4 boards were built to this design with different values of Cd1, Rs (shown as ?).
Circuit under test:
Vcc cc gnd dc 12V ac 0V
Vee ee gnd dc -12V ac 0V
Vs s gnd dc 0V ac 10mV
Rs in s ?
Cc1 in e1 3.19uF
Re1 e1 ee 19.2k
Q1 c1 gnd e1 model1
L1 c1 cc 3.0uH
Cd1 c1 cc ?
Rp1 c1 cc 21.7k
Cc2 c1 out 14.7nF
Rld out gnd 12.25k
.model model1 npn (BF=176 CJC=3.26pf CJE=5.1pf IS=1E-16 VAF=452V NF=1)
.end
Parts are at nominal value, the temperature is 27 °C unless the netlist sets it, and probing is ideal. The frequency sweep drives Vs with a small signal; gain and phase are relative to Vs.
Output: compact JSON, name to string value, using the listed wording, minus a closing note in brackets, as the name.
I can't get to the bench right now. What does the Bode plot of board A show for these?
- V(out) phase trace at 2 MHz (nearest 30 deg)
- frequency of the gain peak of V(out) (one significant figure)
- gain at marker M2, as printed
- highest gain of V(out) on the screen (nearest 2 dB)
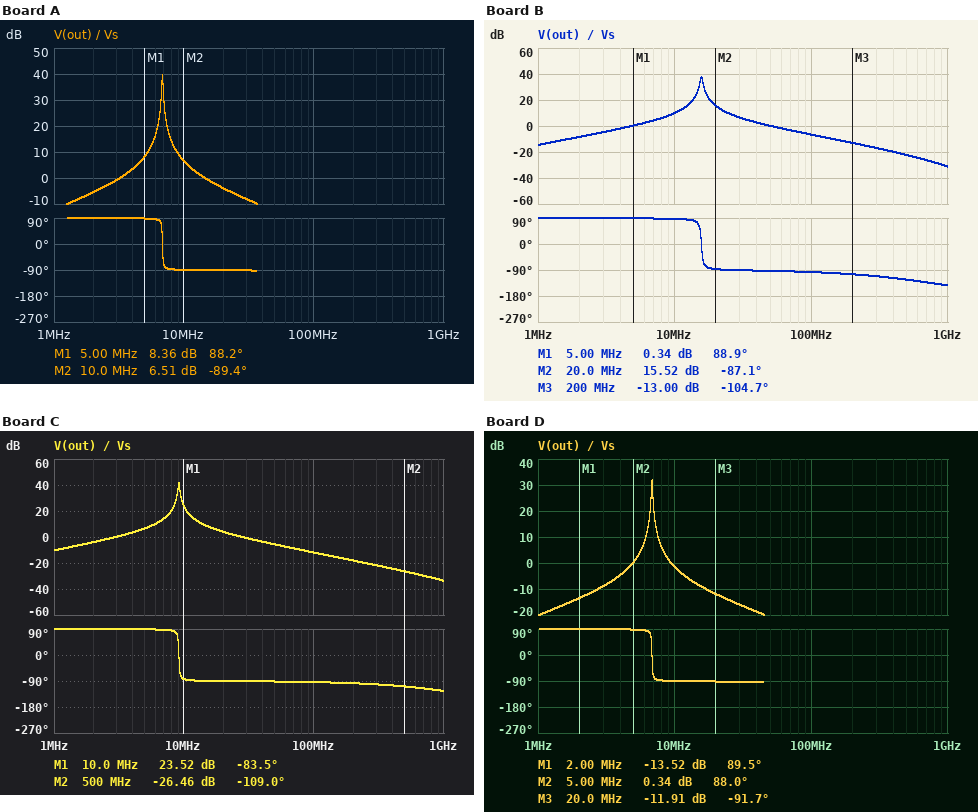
{"V(out) phase trace at 2 MHz": "90 deg", "frequency of the gain peak of V(out)": "7 MHz", "gain at marker M2, as printed": "6.51 dB", "highest gain of V(out) on the screen": "40 dB"}
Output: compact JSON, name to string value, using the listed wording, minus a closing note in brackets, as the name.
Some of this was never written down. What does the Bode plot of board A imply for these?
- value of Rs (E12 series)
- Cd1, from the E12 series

{"value of Rs": "33 Ω", "Cd1, from the E12 series": "180 pF"}
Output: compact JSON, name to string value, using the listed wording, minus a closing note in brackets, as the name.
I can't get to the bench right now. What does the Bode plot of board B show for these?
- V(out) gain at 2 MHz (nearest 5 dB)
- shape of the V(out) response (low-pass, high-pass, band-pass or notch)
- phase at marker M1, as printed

{"V(out) gain at 2 MHz": "-10 dB", "shape of the V(out) response": "band-pass", "phase at marker M1, as printed": "88.9 deg"}
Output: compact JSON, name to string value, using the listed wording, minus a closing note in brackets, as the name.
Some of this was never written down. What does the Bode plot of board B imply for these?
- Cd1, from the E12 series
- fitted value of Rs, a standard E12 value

{"Cd1, from the E12 series": "33 pF", "fitted value of Rs, a standard E12 value": "56 Ω"}
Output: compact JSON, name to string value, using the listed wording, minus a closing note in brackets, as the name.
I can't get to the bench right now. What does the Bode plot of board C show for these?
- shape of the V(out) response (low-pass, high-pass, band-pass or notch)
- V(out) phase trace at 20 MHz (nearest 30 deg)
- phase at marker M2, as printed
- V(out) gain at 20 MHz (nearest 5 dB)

{"shape of the V(out) response": "band-pass", "V(out) phase trace at 20 MHz": "-90 deg", "phase at marker M2, as printed": "-109.0 deg", "V(out) gain at 20 MHz": "5 dB"}
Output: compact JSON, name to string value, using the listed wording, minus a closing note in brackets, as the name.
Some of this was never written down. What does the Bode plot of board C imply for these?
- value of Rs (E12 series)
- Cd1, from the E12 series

{"value of Rs": "18 Ω", "Cd1, from the E12 series": "100 pF"}
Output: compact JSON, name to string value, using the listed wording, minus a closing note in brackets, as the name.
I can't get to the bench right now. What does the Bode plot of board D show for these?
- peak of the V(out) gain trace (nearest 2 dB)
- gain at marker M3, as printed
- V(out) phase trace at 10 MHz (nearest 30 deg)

{"peak of the V(out) gain trace": "32 dB", "gain at marker M3, as printed": "-11.91 dB", "V(out) phase trace at 10 MHz": "-90 deg"}
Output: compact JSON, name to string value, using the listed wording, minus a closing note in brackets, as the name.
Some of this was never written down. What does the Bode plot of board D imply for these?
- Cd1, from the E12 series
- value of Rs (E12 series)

{"Cd1, from the E12 series": "180 pF", "value of Rs": "150 Ω"}
